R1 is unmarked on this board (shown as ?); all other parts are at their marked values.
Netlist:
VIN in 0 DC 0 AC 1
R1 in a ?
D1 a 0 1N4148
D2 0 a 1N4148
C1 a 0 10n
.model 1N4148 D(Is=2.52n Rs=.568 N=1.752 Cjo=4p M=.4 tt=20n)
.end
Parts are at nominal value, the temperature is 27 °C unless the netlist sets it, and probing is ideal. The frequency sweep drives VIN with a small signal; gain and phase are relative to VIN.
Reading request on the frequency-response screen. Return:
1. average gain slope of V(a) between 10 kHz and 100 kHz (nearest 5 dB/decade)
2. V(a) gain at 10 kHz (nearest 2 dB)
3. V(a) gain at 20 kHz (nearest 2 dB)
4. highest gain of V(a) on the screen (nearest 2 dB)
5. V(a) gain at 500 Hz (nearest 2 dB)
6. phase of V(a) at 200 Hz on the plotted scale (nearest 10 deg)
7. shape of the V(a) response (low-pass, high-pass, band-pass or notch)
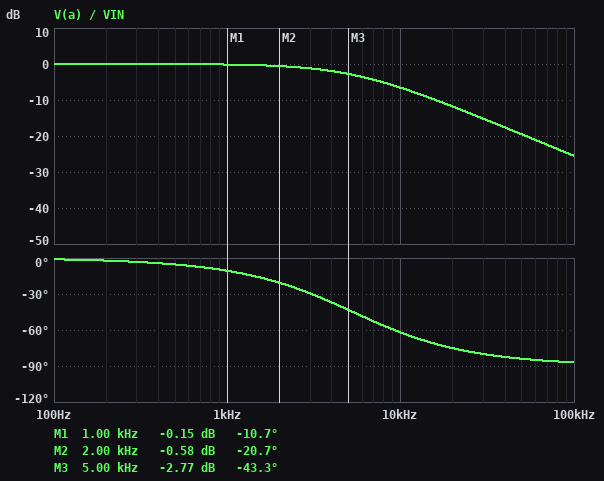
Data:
-20 dB/decade
-6 dB
-12 dB
0 dB
0 dB
0 deg
low-pass
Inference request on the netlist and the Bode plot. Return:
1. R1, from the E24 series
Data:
3 kΩ
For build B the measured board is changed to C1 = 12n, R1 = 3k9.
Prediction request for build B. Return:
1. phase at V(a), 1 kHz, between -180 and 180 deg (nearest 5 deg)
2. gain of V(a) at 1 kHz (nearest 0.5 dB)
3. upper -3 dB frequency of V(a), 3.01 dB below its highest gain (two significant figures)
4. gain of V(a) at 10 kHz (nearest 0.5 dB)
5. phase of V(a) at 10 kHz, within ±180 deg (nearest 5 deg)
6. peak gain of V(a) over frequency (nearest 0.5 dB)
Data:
-15 deg
-0.5 dB
3.4 kHz
-10.0 dB
-70 deg
0 dB
